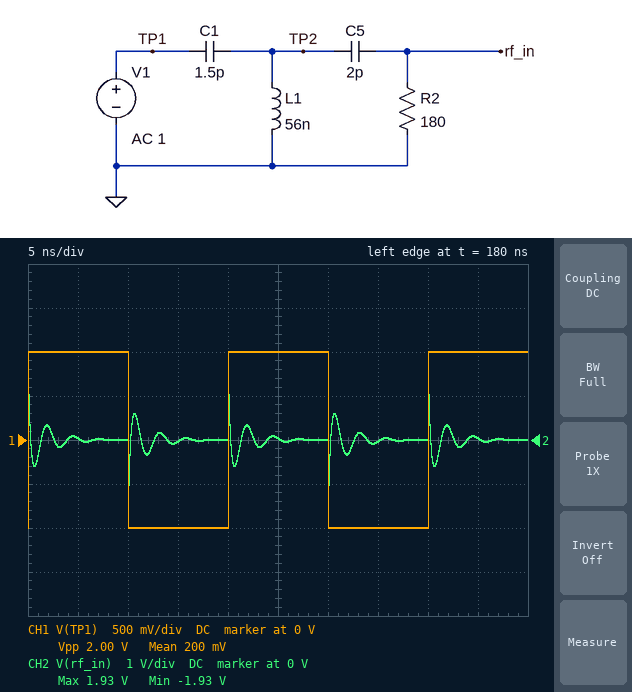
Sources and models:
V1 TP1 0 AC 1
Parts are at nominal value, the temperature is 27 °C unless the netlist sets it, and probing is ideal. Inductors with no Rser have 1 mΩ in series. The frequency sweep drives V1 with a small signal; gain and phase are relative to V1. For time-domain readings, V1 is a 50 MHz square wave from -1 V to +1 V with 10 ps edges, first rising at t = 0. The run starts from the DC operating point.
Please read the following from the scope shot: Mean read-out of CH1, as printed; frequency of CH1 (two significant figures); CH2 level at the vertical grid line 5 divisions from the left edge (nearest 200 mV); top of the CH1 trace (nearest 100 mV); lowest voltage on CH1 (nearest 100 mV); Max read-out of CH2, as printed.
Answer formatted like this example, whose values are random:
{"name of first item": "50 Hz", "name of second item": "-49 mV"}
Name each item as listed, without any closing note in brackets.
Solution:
{"Mean read-out of CH1, as printed": "200 mV", "frequency of CH1": "50 MHz", "CH2 level at the vertical grid line 5 divisions from the left edge": "0 V", "top of the CH1 trace": "1.0 V", "lowest voltage on CH1": "-1.0 V", "Max read-out of CH2, as printed": "1.93 V"}
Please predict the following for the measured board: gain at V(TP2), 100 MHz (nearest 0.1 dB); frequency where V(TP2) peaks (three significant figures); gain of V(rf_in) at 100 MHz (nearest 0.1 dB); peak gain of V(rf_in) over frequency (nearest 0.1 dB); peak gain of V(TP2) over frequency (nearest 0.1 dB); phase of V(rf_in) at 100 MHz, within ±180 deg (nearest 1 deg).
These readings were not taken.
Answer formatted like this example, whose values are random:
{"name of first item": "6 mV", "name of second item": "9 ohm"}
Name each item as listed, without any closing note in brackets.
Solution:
{"gain at V(TP2), 100 MHz": "-28.9 dB", "frequency where V(TP2) peaks": "420 MHz", "gain of V(rf_in) at 100 MHz": "-42.0 dB", "peak gain of V(rf_in) over frequency": "0.4 dB", "peak gain of V(TP2) over frequency": "3.5 dB", "phase of V(rf_in) at 100 MHz, within ±180 deg": "-103 deg"}
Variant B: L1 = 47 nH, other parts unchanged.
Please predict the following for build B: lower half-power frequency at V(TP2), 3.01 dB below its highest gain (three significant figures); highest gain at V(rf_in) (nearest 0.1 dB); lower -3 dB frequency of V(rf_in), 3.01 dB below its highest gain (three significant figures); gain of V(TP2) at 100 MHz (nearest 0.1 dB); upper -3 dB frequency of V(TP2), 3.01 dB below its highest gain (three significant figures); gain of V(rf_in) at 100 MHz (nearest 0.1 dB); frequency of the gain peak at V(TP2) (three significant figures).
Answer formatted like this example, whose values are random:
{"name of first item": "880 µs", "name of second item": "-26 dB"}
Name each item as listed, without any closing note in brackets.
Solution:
{"lower half-power frequency at V(TP2), 3.01 dB below its highest gain": "385 MHz", "highest gain at V(rf_in)": "0.9 dB", "lower -3 dB frequency of V(rf_in), 3.01 dB below its highest gain": "397 MHz", "gain of V(TP2) at 100 MHz": "-30.5 dB", "upper -3 dB frequency of V(TP2), 3.01 dB below its highest gain": "804 MHz", "gain of V(rf_in) at 100 MHz": "-43.7 dB", "frequency of the gain peak at V(TP2)": "472 MHz"}
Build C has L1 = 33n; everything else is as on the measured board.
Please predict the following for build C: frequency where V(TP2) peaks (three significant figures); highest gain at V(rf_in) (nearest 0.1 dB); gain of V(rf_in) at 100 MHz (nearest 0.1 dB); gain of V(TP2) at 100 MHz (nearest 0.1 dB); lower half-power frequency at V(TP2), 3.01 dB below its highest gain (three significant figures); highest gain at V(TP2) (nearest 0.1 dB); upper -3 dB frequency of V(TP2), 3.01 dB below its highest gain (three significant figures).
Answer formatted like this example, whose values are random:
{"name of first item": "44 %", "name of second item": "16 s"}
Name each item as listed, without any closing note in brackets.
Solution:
{"frequency where V(TP2) peaks": "602 MHz", "highest gain at V(rf_in)": "2.1 dB", "gain of V(rf_in) at 100 MHz": "-46.9 dB", "gain of V(TP2) at 100 MHz": "-33.8 dB", "lower half-power frequency at V(TP2), 3.01 dB below its highest gain": "480 MHz", "highest gain at V(TP2)": "3.9 dB", "upper -3 dB frequency of V(TP2), 3.01 dB below its highest gain": "1.15 GHz"}
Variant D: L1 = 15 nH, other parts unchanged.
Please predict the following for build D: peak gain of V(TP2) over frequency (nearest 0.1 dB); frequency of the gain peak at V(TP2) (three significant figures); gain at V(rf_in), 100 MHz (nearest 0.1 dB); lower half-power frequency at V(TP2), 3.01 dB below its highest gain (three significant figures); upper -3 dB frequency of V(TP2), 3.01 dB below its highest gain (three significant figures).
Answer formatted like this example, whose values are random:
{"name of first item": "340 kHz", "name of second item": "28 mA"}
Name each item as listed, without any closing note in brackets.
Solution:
{"peak gain of V(TP2) over frequency": "6.0 dB", "frequency of the gain peak at V(TP2)": "997 MHz", "gain at V(rf_in), 100 MHz": "-54.0 dB", "lower half-power frequency at V(TP2), 3.01 dB below its highest gain": "804 MHz", "upper -3 dB frequency of V(TP2), 3.01 dB below its highest gain": "1.51 GHz"}
